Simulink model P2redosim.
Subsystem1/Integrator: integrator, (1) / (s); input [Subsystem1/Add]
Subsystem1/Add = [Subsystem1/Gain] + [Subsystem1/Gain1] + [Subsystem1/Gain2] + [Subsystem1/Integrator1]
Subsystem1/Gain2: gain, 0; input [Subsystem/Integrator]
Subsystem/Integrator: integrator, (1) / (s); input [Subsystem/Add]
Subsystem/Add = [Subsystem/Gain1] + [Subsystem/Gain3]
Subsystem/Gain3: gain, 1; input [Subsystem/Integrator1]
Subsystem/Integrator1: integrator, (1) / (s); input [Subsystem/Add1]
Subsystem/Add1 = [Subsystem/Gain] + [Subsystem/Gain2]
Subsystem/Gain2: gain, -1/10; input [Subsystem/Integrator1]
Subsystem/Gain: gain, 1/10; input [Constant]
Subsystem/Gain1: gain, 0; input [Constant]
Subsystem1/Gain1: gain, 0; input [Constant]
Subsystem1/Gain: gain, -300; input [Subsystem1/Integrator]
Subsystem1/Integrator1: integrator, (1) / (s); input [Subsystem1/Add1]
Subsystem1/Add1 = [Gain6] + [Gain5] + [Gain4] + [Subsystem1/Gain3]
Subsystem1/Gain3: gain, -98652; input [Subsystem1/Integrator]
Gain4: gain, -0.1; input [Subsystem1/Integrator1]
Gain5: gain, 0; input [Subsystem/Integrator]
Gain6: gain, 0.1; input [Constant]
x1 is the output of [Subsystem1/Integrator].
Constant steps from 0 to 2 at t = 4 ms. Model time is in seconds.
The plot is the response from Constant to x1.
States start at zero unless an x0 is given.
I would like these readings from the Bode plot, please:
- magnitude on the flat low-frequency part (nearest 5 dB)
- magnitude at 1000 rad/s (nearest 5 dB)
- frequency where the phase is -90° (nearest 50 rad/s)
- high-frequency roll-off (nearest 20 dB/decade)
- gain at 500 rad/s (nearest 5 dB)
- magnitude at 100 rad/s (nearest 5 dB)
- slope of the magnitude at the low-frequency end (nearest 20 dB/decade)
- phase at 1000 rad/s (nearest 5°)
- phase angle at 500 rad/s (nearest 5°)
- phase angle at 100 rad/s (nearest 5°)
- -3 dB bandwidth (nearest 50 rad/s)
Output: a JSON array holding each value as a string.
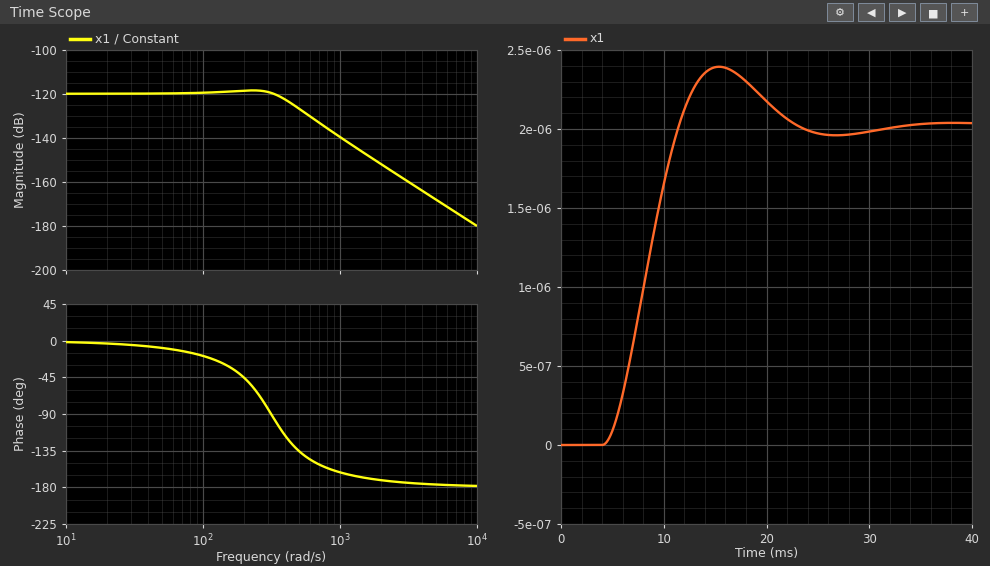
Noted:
["-120 dB", "-140 dB", "300 rad/s", "-40 dB/decade", "-125 dB", "-120 dB", "0 dB/decade", "-160°", "-135°", "-20°", "400 rad/s"]
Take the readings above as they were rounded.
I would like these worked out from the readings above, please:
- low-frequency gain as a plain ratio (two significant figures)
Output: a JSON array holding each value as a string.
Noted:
["0.0000010"]
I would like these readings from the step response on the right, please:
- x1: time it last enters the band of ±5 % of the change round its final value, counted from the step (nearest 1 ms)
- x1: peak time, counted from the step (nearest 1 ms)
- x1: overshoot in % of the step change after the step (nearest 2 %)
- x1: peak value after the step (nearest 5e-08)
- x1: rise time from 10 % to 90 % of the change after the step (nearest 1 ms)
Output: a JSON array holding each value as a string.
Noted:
["17 ms", "11 ms", "18 %", "0.00000240", "5 ms"]
